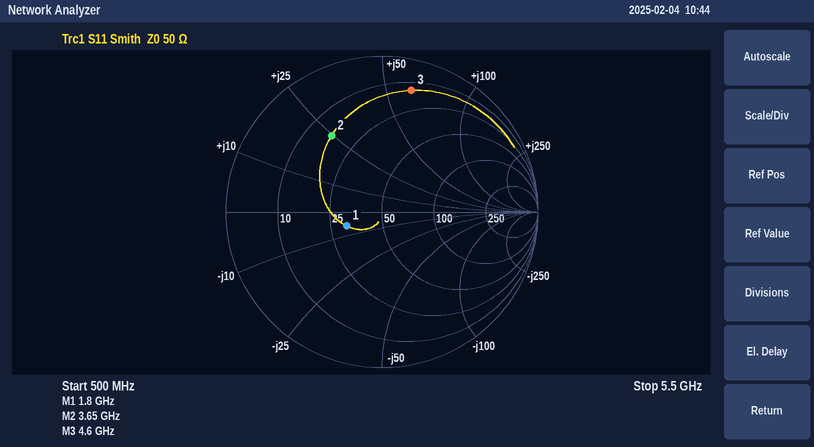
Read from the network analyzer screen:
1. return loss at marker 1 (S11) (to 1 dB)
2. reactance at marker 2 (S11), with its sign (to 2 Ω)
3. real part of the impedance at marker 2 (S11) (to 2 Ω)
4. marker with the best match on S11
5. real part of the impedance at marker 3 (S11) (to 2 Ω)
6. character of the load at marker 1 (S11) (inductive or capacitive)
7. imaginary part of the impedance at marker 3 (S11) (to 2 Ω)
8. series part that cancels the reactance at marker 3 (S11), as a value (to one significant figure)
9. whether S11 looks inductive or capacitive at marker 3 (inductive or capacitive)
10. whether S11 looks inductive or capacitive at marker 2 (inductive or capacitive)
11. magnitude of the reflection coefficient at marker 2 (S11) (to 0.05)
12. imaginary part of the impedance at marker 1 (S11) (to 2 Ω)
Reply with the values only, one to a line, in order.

12 dB
+24 Ω
16 Ω
marker 1
14 Ω
capacitive
+62 Ω
600 fF
inductive
inductive
0.60
-6 Ω
